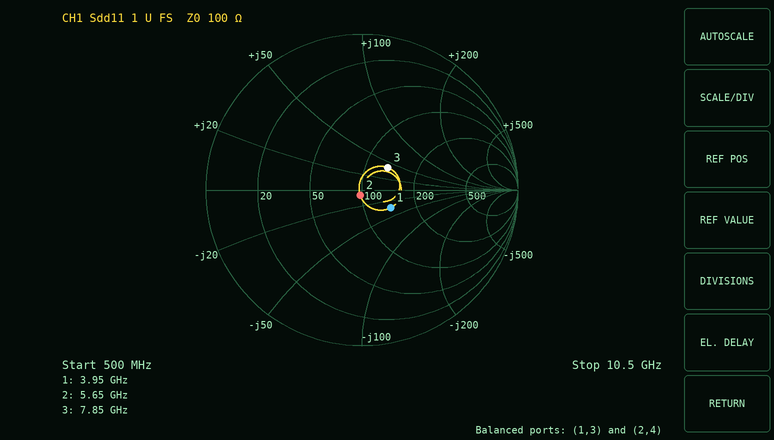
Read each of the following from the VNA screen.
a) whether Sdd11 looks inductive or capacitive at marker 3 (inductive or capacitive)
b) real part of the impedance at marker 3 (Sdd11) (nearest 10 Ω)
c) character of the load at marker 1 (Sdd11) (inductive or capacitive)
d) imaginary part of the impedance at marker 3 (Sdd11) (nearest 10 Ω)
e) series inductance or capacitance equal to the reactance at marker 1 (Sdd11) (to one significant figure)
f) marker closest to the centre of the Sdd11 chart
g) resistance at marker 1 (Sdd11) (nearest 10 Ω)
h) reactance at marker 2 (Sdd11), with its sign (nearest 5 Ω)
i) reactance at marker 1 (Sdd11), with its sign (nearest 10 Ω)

inductive
130 Ω
capacitive
+40 Ω
1 pF
marker 2
140 Ω
-5 Ω
-30 Ω
